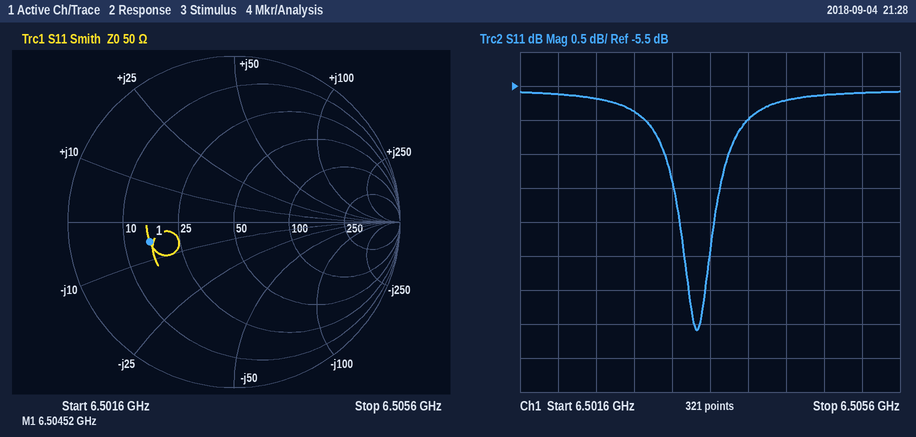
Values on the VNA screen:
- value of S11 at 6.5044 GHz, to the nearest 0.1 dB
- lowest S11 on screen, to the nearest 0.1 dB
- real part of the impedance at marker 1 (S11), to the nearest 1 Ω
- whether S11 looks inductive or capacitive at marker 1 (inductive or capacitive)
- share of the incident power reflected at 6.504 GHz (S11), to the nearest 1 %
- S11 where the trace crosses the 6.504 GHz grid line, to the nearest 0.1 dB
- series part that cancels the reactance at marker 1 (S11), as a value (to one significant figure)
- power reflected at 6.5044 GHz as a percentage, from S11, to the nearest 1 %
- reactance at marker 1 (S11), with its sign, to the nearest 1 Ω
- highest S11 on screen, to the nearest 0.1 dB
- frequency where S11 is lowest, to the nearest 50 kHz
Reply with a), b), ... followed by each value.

a) -5.7 dB
b) -9.1 dB
c) 16 Ω
d) capacitive
e) 25 %
f) -6.0 dB
g) 100 pH
h) 27 %
i) -5 Ω
j) -5.6 dB
k) 6.50345 GHz
